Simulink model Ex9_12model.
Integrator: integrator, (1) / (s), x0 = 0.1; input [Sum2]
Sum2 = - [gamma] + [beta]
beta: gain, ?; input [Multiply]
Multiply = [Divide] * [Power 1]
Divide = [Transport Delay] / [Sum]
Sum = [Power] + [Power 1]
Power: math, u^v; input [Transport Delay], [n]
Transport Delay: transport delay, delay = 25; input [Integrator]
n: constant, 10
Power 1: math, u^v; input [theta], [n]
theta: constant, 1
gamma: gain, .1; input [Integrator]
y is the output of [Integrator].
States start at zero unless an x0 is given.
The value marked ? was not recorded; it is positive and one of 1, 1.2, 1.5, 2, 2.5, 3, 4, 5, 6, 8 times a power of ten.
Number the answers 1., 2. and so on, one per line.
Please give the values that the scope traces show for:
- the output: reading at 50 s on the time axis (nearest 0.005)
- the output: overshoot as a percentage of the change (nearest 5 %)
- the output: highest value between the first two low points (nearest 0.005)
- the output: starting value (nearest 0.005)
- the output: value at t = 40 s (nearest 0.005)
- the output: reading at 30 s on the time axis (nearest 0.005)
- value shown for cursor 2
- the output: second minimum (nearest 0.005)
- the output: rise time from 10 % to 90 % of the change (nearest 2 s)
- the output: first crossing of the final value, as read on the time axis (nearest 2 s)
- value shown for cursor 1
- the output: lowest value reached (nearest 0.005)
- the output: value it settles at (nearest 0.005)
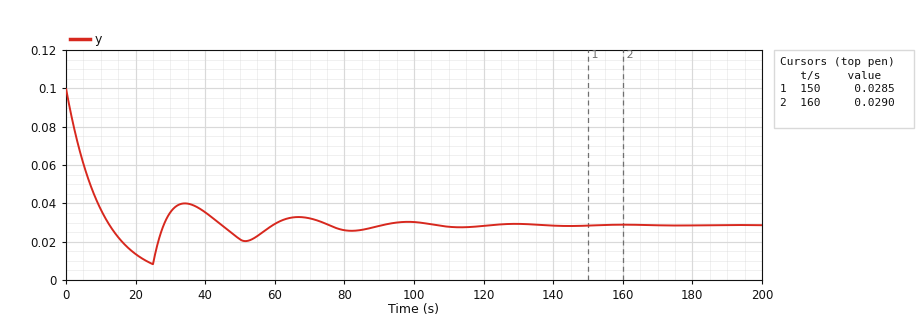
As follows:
1. 0.020
2. 30 %
3. 0.040
4. 0.100
5. 0.035
6. 0.035
7. 0.0290
8. 0.020
9. 10 s
10. 12 s
11. 0.0285
12. 0.010
13. 0.030
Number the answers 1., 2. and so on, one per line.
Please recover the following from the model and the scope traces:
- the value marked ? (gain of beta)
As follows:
1. 0.1
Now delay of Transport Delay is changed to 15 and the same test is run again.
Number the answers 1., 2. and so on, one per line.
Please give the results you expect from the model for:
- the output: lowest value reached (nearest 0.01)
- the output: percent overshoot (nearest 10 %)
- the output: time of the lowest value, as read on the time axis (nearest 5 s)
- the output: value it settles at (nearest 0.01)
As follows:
1. 0.02
2. 30 %
3. 15 s
4. 0.04
